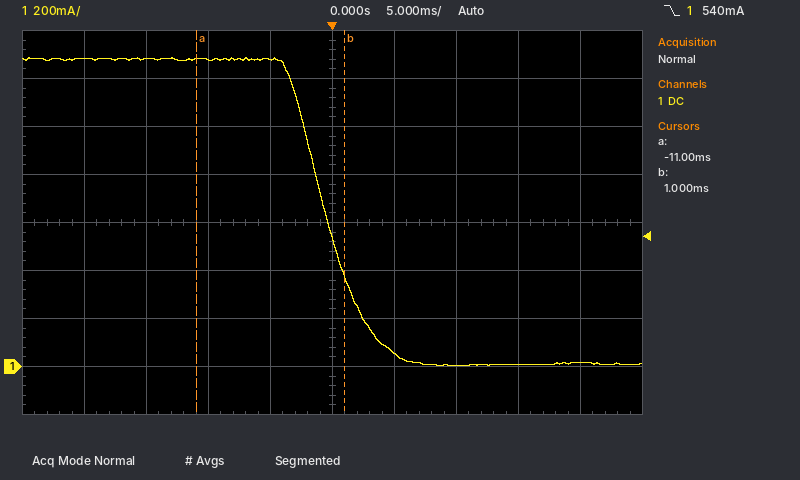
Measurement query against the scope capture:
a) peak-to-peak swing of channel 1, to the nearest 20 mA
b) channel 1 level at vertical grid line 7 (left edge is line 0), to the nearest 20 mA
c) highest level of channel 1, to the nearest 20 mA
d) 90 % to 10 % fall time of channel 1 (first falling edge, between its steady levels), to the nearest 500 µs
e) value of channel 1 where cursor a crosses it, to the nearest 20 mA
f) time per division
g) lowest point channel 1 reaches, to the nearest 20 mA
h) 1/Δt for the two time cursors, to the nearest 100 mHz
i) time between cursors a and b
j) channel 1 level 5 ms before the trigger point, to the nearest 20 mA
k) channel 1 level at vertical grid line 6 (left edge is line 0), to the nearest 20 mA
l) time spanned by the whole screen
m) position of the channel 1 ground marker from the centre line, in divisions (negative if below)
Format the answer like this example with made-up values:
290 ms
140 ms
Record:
1.28 A
0 mA
1.28 A
6.5 ms
1.28 A
5 ms
0 mA
83.3 Hz
12.0 ms
1.28 A
60 mA
50 ms
-3.0 div
